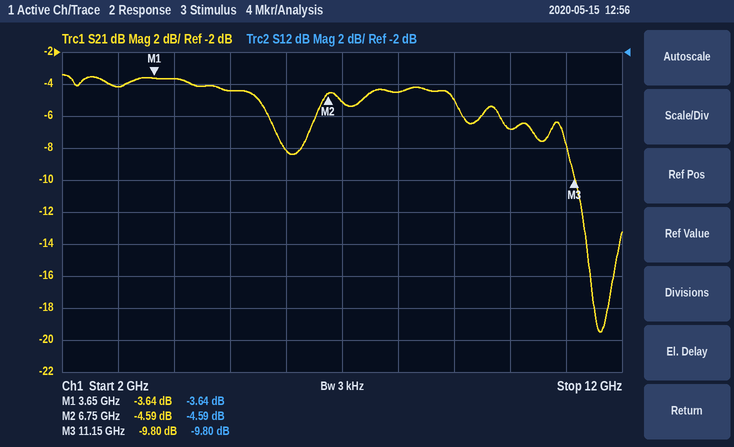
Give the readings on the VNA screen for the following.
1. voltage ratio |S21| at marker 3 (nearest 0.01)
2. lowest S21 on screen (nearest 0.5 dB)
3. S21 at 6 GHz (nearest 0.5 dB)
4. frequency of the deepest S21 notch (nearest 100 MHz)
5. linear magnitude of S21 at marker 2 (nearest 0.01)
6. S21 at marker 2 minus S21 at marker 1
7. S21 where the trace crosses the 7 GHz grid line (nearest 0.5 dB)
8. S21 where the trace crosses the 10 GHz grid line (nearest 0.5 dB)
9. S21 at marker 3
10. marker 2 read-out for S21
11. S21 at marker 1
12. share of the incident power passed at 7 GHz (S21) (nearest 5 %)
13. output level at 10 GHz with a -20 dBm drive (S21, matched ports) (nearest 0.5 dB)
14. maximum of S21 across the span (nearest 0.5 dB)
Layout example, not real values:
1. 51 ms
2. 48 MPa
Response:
1. 0.32
2. -19.5 dB
3. -8.0 dB
4. 11.6 GHz
5. 0.59
6. -0.95 dB
7. -5.0 dB
8. -7.0 dB
9. -9.80 dB
10. -4.59 dB
11. -3.64 dB
12. 30 %
13. -27.0 dBm
14. -3.5 dB
